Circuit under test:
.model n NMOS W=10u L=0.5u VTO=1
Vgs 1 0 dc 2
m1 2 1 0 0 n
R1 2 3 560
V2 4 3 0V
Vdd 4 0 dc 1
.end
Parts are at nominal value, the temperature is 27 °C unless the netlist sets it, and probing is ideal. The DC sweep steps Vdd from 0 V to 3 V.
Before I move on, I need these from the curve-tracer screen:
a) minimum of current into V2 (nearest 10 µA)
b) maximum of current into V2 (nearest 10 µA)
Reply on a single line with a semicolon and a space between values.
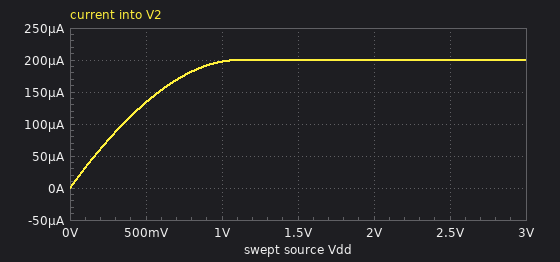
0 A; 200 µA
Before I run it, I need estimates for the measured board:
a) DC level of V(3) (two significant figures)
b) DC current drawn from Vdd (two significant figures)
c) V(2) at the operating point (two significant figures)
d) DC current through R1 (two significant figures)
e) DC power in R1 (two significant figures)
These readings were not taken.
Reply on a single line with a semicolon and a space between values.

1.0 V; 200 µA; 890 mV; 200 µA; 22 µW
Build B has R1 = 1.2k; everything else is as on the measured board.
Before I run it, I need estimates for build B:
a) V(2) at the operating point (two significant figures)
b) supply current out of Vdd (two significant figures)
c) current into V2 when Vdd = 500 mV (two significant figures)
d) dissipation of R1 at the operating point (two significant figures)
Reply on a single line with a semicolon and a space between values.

770 mV; 190 µA; 120 µA; 43 µW
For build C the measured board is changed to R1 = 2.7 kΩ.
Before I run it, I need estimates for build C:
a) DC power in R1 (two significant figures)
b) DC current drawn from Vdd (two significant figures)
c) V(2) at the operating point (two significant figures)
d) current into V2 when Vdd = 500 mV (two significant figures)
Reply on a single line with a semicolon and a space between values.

71 µW; 160 µA; 560 mV; 90 µA
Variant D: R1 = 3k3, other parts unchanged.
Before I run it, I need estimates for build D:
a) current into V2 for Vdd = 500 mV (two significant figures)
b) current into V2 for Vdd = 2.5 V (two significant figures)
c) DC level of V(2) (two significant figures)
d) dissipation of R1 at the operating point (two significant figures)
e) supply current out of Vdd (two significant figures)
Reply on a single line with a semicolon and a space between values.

82 µA; 200 µA; 500 mV; 75 µW; 150 µA
